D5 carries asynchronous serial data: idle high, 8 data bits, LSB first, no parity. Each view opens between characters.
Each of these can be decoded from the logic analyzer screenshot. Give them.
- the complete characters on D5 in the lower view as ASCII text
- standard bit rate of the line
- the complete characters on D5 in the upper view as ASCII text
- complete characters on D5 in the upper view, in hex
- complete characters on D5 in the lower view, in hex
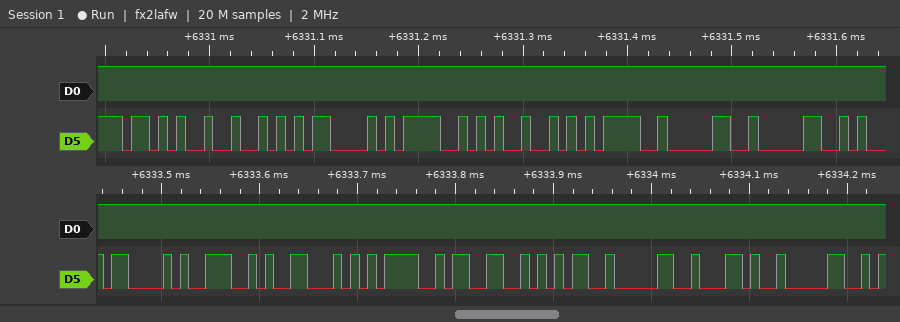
"CNF=350,0"
115200 baud
"+RCOI=00"
2B, 52, 43, 4F, 49, 3D, 30, 30
43, 4E, 46, 3D, 33, 35, 30, 2C, 30
